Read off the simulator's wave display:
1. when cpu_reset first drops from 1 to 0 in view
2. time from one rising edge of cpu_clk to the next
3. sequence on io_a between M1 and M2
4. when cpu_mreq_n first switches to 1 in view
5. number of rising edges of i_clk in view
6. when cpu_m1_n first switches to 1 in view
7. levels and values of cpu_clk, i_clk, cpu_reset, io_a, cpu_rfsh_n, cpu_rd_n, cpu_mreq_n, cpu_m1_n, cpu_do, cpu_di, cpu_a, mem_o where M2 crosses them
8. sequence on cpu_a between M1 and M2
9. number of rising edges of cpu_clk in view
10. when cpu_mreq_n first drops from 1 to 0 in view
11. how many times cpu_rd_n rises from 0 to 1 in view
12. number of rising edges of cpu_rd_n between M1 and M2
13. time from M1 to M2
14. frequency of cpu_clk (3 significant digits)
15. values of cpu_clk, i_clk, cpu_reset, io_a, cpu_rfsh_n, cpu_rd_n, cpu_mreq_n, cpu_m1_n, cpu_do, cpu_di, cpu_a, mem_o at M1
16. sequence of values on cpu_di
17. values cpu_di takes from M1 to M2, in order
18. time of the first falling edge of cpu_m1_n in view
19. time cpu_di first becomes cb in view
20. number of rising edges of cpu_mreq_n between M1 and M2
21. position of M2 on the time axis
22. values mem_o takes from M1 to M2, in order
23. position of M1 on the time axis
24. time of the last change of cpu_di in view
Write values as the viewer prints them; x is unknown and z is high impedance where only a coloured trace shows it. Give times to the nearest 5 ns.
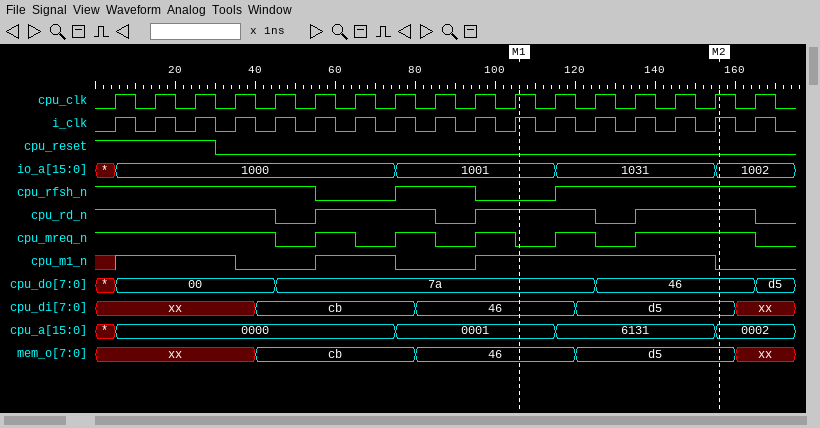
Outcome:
30 ns
10 ns
1001, 1031, 1002
55 ns
17
5 ns
cpu_clk=1, i_clk=1, cpu_reset=0, io_a=1002, cpu_rfsh_n=1, cpu_rd_n=1, cpu_mreq_n=1, cpu_m1_n=0, cpu_do=46, cpu_di=d5, cpu_a=0002, mem_o=d5
0001, 6131, 0002
17
45 ns
3
1
50 ns
100 MHz
cpu_clk=1, i_clk=1, cpu_reset=0, io_a=1001, cpu_rfsh_n=0, cpu_rd_n=1, cpu_mreq_n=0, cpu_m1_n=1, cpu_do=7a, cpu_di=46, cpu_a=0001, mem_o=46
xx, cb, 46, d5, xx
46, d5
35 ns
40 ns
2
155 ns
46, d5
105 ns
160 ns
